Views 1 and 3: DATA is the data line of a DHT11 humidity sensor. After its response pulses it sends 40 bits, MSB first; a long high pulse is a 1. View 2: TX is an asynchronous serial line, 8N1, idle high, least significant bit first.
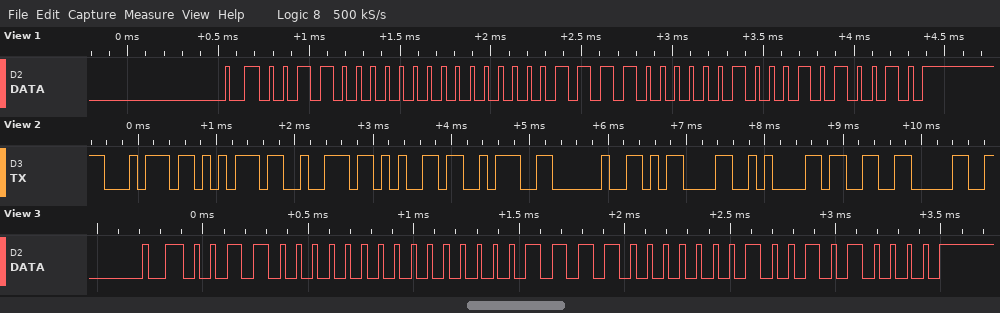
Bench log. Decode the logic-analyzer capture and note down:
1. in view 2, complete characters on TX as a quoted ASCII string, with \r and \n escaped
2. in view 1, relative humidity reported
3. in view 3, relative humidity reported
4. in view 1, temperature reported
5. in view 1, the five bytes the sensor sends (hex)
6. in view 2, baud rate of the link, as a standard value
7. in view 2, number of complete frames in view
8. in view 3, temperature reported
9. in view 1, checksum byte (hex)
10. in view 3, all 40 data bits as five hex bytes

"ture: \r\n30"
48 %
48 %
30.4 °C
30 00 1E 04 52
9600 baud
10
30.2 °C
0x52
30 00 1E 02 50
